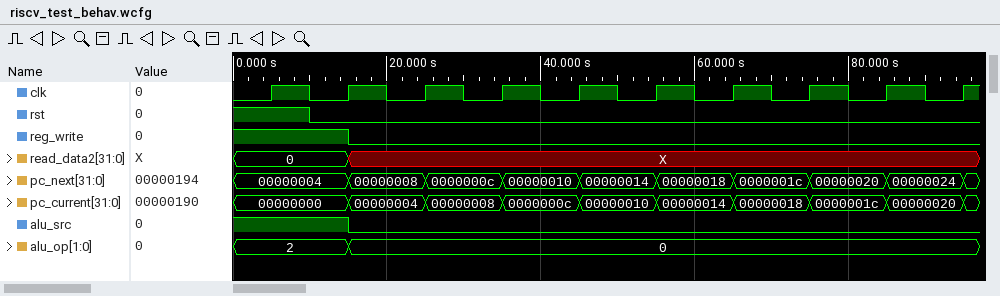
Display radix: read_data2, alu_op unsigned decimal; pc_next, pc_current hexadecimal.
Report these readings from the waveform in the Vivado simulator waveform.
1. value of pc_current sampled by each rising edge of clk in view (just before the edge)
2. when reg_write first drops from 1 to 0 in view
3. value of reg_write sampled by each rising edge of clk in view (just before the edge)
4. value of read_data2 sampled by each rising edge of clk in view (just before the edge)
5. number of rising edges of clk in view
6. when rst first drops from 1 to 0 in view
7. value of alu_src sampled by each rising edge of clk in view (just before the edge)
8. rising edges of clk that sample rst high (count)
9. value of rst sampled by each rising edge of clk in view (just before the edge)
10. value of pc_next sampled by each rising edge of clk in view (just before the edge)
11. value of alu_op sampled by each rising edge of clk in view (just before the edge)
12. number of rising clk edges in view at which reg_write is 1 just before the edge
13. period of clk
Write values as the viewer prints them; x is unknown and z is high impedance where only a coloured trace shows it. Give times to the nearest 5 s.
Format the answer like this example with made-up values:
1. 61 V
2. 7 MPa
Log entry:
1. 00000000, 00000000, 00000004, 00000008, 0000000c, 00000010, 00000014, 00000018, 0000001c, 00000020
2. 15 s
3. 1 1 0 0 0 0 0 0 0 0
4. 0, 0, X, X, X, X, X, X, X, X
5. 10
6. 10 s
7. 1 1 0 0 0 0 0 0 0 0
8. 1
9. 1 0 0 0 0 0 0 0 0 0
10. 00000004, 00000004, 00000008, 0000000c, 00000010, 00000014, 00000018, 0000001c, 00000020, 00000024
11. 2, 2, 0, 0, 0, 0, 0, 0, 0, 0
12. 2
13. 10 s
